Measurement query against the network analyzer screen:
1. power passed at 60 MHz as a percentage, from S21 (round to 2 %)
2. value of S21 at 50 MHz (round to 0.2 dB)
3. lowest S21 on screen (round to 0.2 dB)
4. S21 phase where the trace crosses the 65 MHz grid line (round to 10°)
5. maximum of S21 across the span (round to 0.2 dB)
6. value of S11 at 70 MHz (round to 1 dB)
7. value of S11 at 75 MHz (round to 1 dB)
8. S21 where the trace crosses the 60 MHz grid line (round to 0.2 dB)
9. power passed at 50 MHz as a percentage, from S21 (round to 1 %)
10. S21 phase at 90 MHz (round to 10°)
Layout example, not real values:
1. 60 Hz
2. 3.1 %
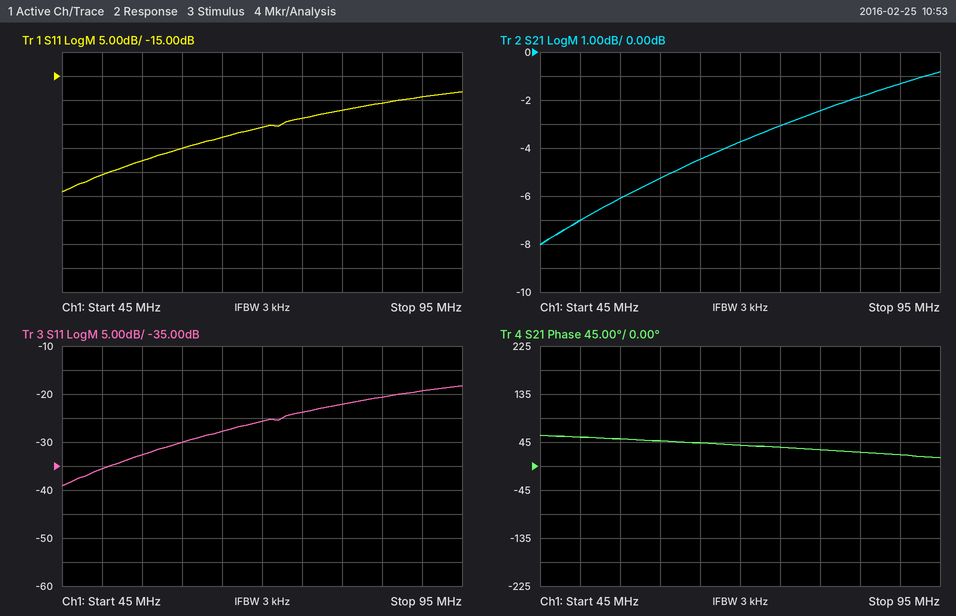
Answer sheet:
1. 30 %
2. -7.0 dB
3. -8.0 dB
4. 40°
5. -0.8 dB
6. -26 dB
7. -24 dB
8. -5.2 dB
9. 20 %
10. 20°
